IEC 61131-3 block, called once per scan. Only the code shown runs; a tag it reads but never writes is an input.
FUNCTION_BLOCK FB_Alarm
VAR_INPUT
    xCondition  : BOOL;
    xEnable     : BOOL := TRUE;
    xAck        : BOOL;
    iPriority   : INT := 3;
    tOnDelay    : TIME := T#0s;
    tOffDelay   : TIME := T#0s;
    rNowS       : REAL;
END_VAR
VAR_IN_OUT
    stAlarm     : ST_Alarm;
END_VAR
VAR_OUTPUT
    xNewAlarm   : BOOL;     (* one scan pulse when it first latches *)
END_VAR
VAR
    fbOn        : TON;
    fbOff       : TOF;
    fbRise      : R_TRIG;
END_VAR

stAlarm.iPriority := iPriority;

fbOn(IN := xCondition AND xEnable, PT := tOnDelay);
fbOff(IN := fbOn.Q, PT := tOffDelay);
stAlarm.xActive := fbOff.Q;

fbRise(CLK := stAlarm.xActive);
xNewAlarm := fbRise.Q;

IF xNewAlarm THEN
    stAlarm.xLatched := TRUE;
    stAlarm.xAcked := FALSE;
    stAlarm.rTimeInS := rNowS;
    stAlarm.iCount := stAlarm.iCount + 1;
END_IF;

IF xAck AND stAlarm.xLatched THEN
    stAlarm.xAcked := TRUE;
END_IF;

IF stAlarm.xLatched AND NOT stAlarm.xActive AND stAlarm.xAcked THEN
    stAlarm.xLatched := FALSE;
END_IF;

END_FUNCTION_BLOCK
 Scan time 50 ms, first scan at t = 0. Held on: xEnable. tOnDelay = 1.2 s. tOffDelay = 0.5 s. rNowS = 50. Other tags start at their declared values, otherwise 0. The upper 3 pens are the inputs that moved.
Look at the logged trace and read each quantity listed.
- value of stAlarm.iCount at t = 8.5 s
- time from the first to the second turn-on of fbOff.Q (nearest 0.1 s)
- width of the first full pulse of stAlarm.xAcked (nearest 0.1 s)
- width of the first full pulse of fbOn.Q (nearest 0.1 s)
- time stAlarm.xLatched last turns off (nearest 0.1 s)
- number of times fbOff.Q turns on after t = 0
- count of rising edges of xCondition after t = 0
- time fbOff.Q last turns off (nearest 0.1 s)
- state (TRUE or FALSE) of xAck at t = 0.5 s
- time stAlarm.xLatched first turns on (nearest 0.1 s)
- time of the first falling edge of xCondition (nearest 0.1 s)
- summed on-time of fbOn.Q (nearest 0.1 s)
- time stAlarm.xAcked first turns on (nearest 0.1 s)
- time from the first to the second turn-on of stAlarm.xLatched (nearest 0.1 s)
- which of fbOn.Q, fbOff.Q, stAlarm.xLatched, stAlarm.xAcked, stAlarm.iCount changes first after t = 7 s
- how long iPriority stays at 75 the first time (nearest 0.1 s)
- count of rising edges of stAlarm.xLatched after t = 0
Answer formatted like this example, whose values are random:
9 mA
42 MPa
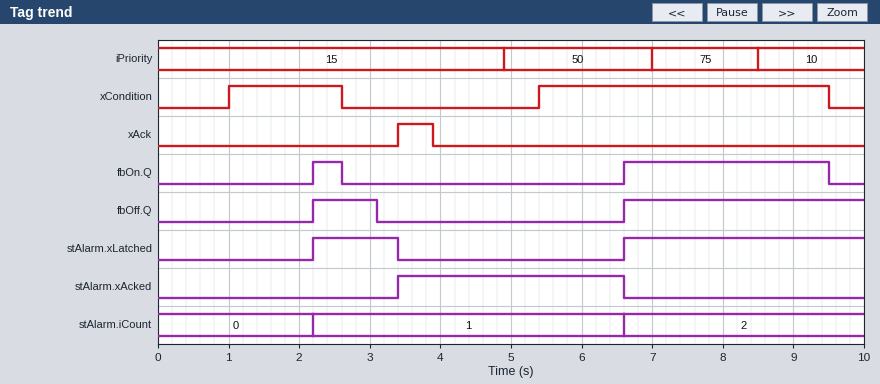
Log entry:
2
4.4 s
3.2 s
0.4 s
3.4 s
2
2
3.1 s
FALSE
2.2 s
2.6 s
3.3 s
3.4 s
4.4 s
fbOn.Q
1.5 s
2
